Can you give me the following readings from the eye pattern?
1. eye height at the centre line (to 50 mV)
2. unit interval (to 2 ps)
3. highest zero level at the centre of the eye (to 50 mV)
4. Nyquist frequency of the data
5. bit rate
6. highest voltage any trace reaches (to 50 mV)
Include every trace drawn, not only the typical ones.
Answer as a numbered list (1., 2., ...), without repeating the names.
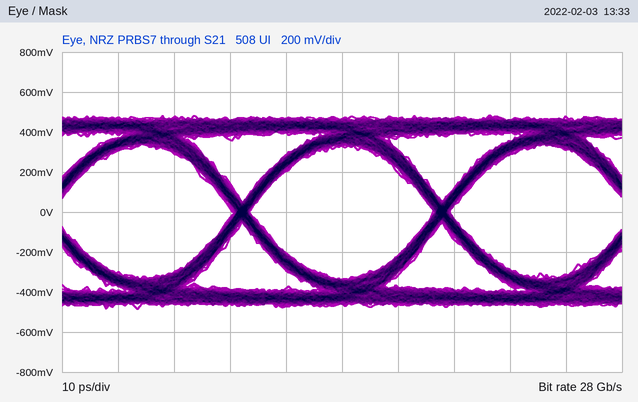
1. 650 mV
2. 36 ps
3. -350 mV
4. 14 GHz
5. 28 Gb/s
6. 500 mV
